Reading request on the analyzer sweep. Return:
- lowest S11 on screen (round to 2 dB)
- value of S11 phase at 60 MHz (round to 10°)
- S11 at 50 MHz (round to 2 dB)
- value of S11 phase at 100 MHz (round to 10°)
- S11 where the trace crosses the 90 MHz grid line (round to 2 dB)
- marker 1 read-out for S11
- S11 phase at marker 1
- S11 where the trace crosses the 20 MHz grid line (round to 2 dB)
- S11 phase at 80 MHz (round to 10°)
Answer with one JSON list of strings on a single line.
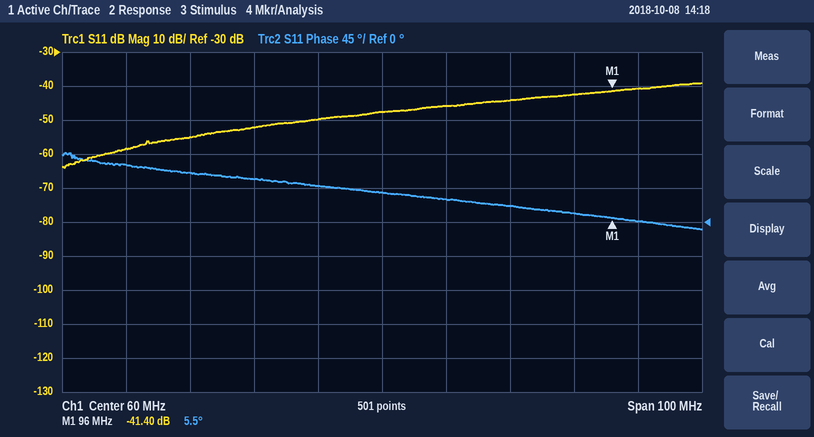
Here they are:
["-64 dB", "40°", "-50 dB", "0°", "-42 dB", "-41.40 dB", "5.5°", "-58 dB", "20°"]
